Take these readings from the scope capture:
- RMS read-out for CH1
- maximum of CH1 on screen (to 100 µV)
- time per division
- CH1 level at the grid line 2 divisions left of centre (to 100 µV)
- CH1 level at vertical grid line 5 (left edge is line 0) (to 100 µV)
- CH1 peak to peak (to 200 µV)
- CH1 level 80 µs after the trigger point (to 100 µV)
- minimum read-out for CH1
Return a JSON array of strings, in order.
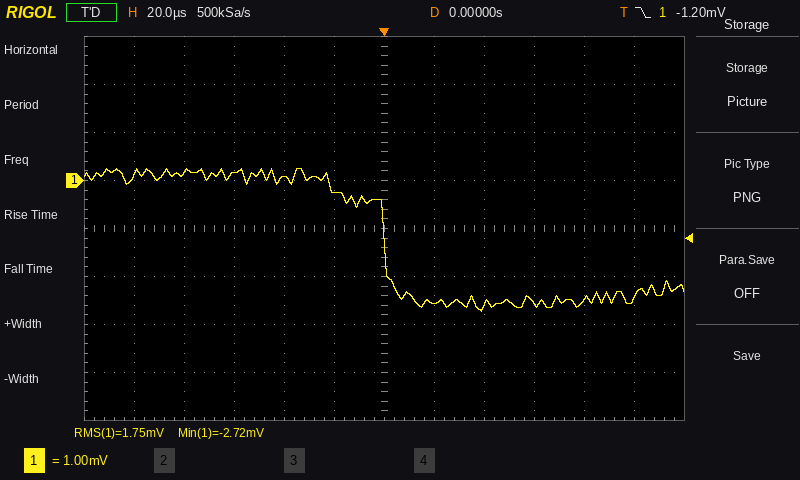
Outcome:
["1.75 mV", "200 µV", "20 µs", "100 µV", "-200 µV", "3.0 mV", "-2.5 mV", "-2.72 mV"]
